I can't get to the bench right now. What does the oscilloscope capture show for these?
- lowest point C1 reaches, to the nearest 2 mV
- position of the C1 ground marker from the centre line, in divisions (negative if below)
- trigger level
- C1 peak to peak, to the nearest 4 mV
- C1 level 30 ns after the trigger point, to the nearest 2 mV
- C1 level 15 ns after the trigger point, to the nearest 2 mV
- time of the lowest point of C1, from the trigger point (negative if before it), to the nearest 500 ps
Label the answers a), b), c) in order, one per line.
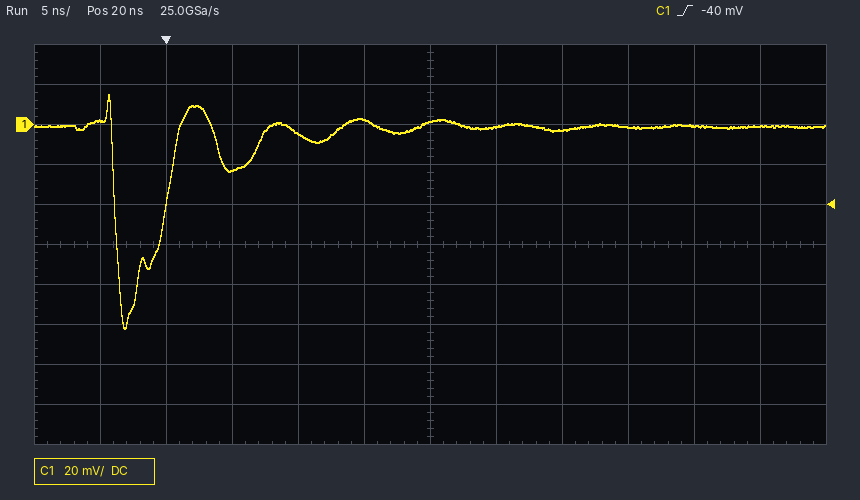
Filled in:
a) -102 mV
b) +3.0 div
c) -40 mV
d) 116 mV
e) -2 mV
f) 2 mV
g) -3.0 ns
